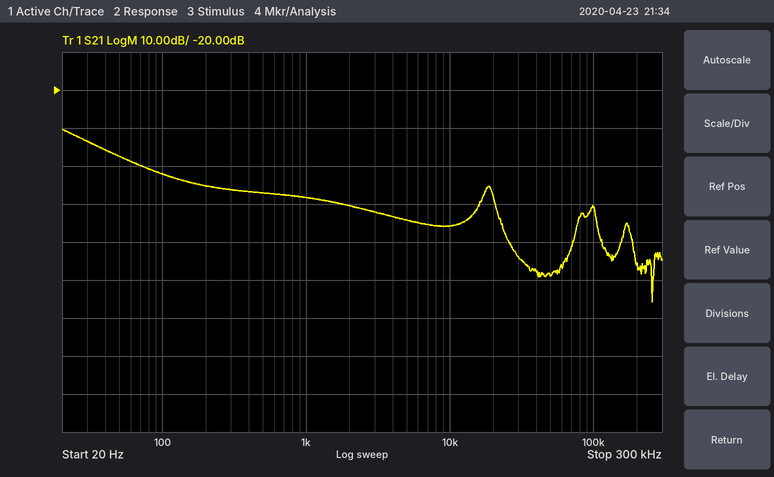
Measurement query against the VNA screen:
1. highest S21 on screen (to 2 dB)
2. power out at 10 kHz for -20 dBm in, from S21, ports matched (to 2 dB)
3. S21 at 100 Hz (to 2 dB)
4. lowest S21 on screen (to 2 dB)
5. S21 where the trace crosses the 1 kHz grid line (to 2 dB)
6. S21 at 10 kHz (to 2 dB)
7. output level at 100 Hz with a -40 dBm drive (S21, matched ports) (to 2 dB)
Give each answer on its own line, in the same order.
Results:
-30 dB
-76 dBm
-42 dB
-76 dB
-48 dB
-56 dB
-82 dBm
